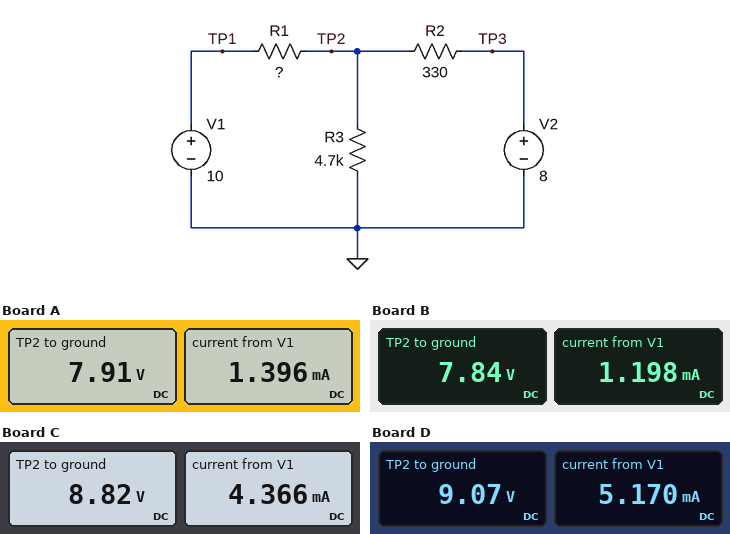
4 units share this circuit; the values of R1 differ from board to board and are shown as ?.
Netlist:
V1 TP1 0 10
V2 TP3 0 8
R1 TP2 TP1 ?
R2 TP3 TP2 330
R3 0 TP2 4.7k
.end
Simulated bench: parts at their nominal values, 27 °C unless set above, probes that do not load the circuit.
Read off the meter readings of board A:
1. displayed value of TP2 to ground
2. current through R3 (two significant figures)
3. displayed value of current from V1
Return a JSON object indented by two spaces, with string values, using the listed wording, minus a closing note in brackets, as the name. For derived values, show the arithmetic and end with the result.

{
  "displayed value of TP2 to ground": "7.91 V",
  "current through R3": "(7.91 V) / 4.7 kΩ = 1.7 mA",
  "displayed value of current from V1": "1.396 mA"
}
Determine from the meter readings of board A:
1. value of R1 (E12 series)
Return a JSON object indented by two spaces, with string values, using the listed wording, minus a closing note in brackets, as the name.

{
  "value of R1": "1.5 kΩ"
}
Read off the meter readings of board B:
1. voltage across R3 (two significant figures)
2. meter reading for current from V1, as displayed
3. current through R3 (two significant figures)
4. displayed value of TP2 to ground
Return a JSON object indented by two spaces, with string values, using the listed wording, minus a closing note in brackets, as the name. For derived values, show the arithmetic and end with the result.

{
  "voltage across R3": "7.84 V = 7.8 V",
  "meter reading for current from V1, as displayed": "1.198 mA",
  "current through R3": "(7.84 V) / 4.7 kΩ = 1.7 mA",
  "displayed value of TP2 to ground": "7.84 V"
}
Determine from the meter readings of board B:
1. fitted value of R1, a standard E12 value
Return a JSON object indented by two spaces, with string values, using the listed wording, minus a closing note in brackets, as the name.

{
  "fitted value of R1, a standard E12 value": "1.8 kΩ"
}
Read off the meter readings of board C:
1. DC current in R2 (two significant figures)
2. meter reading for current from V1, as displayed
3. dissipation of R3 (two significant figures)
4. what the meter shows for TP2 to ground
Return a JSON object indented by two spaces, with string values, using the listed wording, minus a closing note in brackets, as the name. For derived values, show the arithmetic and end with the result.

{
  "DC current in R2": "(8.82 V - 8 V) / 330 Ω = 2.5 mA",
  "meter reading for current from V1, as displayed": "4.366 mA",
  "dissipation of R3": "(8.82 V)^2 / 4.7 kΩ = 17 mW",
  "what the meter shows for TP2 to ground": "8.82 V"
}
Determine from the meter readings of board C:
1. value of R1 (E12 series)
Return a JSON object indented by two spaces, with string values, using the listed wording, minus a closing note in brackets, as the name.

{
  "value of R1": "270 Ω"
}
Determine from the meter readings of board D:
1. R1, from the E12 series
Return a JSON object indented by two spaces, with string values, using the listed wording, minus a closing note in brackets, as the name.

{
  "R1, from the E12 series": "180 Ω"
}
